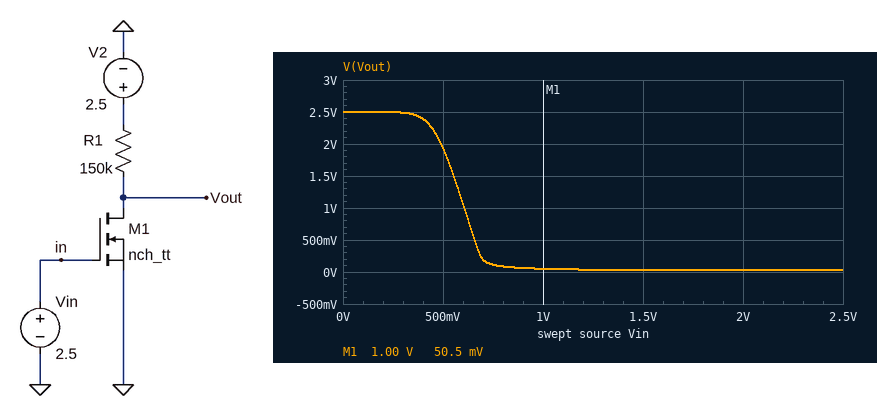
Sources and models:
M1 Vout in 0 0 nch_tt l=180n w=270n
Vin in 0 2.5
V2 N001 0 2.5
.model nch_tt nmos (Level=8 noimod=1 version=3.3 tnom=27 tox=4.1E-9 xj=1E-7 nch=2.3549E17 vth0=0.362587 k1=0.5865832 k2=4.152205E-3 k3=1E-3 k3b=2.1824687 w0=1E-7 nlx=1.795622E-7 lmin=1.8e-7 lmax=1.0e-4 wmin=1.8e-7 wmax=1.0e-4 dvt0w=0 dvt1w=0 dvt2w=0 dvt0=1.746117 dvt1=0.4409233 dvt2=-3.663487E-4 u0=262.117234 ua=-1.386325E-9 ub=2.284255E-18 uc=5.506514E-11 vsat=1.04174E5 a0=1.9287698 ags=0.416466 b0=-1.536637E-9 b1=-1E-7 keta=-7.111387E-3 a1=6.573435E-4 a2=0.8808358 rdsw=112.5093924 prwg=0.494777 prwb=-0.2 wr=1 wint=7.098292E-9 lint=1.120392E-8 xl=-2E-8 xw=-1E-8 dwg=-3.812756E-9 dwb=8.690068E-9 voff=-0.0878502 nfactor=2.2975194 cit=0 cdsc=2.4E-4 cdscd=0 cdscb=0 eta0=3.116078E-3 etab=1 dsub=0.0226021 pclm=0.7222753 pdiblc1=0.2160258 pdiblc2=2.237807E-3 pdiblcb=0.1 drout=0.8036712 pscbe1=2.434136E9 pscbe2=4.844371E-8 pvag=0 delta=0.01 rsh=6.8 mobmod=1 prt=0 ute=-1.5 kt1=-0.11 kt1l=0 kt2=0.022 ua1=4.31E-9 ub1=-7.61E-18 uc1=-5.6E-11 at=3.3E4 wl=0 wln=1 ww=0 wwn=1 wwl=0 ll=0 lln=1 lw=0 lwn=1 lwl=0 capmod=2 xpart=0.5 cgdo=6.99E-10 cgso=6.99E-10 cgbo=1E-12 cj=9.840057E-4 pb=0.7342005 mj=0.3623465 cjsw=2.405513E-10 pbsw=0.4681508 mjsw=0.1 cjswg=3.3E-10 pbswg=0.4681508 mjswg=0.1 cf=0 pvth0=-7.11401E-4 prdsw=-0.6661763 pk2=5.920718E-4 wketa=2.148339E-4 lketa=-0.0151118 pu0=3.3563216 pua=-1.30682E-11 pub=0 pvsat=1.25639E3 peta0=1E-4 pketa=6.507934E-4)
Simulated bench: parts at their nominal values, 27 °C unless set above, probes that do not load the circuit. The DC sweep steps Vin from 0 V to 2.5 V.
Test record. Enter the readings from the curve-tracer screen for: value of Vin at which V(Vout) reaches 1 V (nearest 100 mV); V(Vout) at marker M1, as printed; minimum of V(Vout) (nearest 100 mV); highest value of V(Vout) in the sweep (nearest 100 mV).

600 mV
50.5 mV
0 V
2.5 V
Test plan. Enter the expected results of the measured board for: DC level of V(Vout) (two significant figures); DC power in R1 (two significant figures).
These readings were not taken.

26 mV
41 µW
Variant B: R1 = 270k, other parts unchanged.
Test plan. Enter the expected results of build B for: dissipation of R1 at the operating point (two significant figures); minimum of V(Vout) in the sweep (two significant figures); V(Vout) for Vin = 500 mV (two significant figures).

23 µW
14 mV
1.6 V
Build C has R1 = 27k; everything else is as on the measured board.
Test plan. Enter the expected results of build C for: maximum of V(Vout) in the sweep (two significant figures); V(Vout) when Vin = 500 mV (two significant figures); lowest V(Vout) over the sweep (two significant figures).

2.5 V
2.4 V
150 mV
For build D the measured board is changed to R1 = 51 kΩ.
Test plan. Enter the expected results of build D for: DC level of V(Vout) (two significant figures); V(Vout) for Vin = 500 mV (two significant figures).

78 mV
2.3 V
